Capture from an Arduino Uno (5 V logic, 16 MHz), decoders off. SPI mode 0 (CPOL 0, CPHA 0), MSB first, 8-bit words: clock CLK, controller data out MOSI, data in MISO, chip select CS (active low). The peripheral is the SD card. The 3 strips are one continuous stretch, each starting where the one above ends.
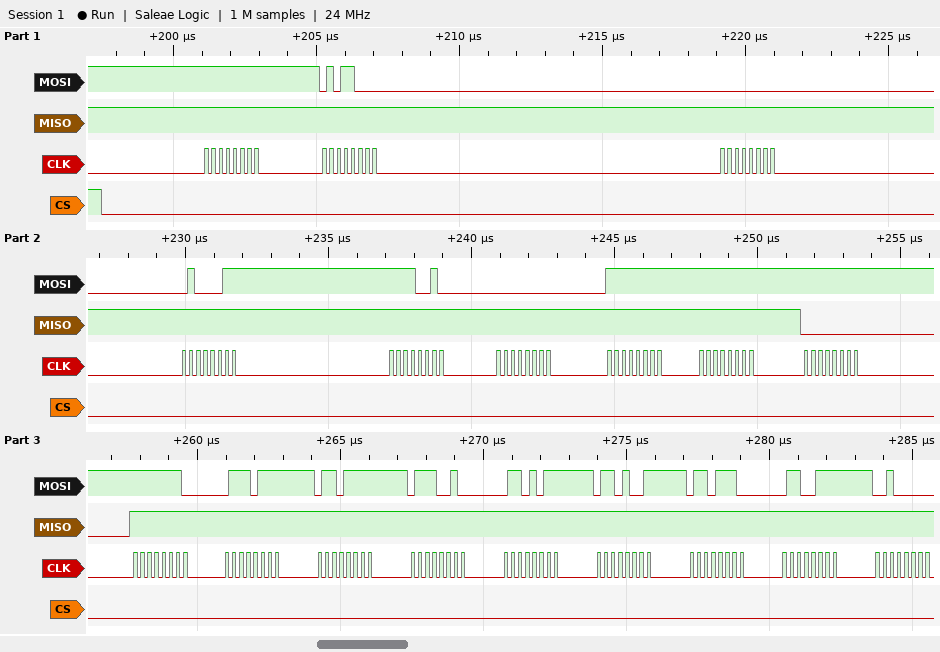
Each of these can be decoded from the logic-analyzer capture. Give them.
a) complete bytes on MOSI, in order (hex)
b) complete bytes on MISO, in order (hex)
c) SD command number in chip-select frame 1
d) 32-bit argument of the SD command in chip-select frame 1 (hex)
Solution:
0xFF 0x58 0x00 0x43 0xF2 0x00 0xFF 0xFF 0xFF 0xFE 0x77 0x6F 0x72 0x6B 0x69 0x6E 0x67 0x20
0xFF 0xFF 0xFF 0xFF 0xFF 0xFF 0xFF 0xFF 0x00 0xFF 0xFF 0xFF 0xFF 0xFF 0xFF 0xFF 0xFF 0xFF
CMD24
0x0043F200
